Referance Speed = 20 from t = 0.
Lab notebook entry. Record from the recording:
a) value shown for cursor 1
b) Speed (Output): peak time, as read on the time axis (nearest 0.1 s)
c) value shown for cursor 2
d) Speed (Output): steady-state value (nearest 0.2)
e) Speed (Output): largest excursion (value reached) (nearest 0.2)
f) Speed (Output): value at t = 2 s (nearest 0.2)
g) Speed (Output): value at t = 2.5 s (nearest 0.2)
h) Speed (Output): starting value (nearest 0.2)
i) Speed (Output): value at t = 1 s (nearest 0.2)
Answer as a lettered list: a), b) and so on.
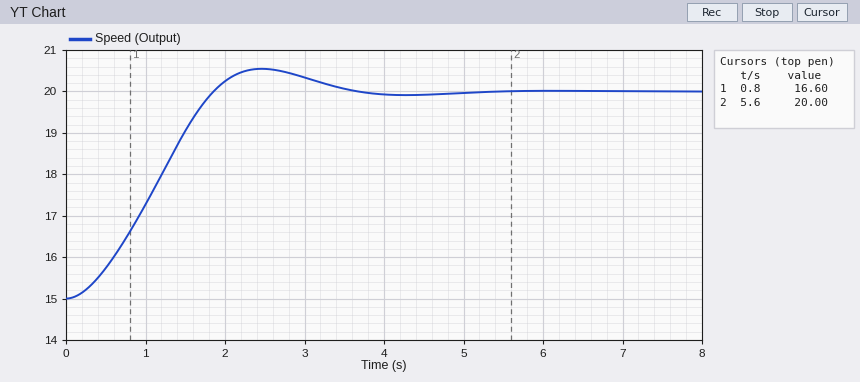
a) 16.60
b) 2.5 s
c) 20.00
d) 20.0
e) 20.6
f) 20.2
g) 20.6
h) 15.0
i) 17.2
